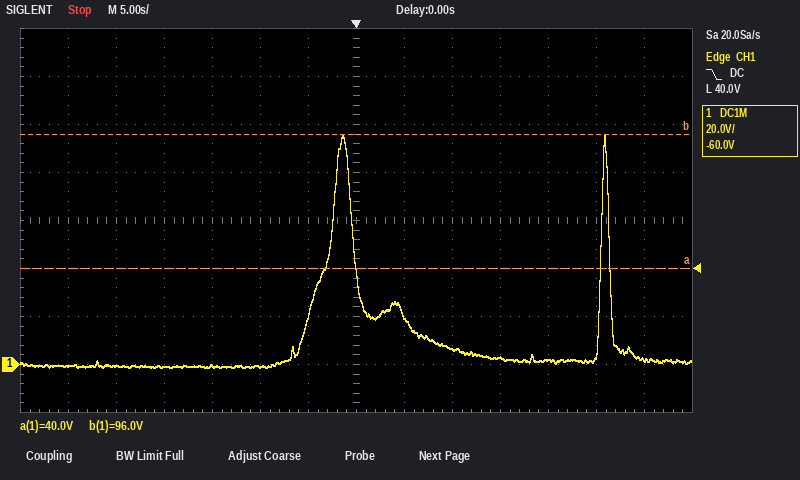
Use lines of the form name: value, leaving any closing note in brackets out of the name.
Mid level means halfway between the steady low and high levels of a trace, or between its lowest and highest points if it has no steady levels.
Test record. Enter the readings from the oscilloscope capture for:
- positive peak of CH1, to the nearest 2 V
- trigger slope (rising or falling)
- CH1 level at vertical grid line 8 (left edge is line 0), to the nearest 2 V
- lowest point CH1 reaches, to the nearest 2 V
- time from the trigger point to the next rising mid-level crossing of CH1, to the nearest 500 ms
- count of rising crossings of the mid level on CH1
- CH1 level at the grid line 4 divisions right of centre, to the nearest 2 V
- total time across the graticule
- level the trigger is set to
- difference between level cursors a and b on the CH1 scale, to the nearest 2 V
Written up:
positive peak of CH1, to the nearest 2 V: 96 V
trigger slope: falling
CH1 level at vertical grid line 8 (left edge is line 0), to the nearest 2 V: 20 V
lowest point CH1 reaches, to the nearest 2 V: -2 V
time from the trigger point to the next rising mid-level crossing of CH1, to the nearest 500 ms: 25.5 s
count of rising crossings of the mid level on CH1: 2
CH1 level at the grid line 4 divisions right of centre, to the nearest 2 V: 2 V
total time across the graticule: 70 s
level the trigger is set to: 40.0 V
difference between level cursors a and b on the CH1 scale, to the nearest 2 V: 56 V
